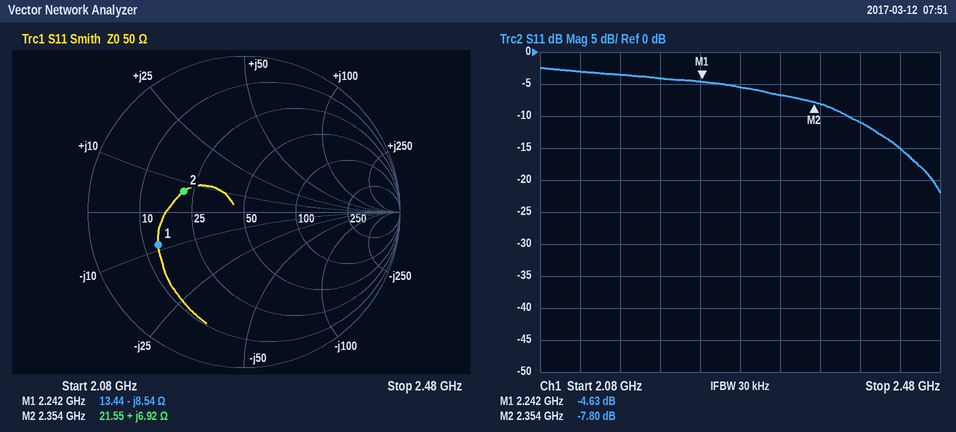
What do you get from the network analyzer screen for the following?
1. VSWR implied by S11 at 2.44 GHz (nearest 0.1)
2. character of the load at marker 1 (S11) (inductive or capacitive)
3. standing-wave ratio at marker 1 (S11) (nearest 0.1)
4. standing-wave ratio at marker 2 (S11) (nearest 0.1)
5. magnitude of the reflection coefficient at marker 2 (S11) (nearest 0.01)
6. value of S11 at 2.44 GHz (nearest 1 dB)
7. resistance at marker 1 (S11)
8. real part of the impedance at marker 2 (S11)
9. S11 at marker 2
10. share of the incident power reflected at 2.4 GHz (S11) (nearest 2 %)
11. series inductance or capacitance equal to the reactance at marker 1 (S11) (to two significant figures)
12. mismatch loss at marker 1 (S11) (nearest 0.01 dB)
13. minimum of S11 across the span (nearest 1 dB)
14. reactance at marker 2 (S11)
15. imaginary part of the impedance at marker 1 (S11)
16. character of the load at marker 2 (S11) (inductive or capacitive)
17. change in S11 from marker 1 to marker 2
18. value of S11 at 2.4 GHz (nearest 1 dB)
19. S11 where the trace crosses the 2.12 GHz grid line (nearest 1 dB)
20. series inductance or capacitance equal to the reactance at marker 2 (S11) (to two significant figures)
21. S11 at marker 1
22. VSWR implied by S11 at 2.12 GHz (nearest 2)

1.4
capacitive
3.8
2.4
0.41
-15 dB
13.44 Ω
21.55 Ω
-7.80 dB
8 %
8.3 pF
1.83 dB
-22 dB
+6.92 Ω
-8.54 Ω
inductive
-3.17 dB
-11 dB
-3 dB
470 pH
-4.63 dB
6
